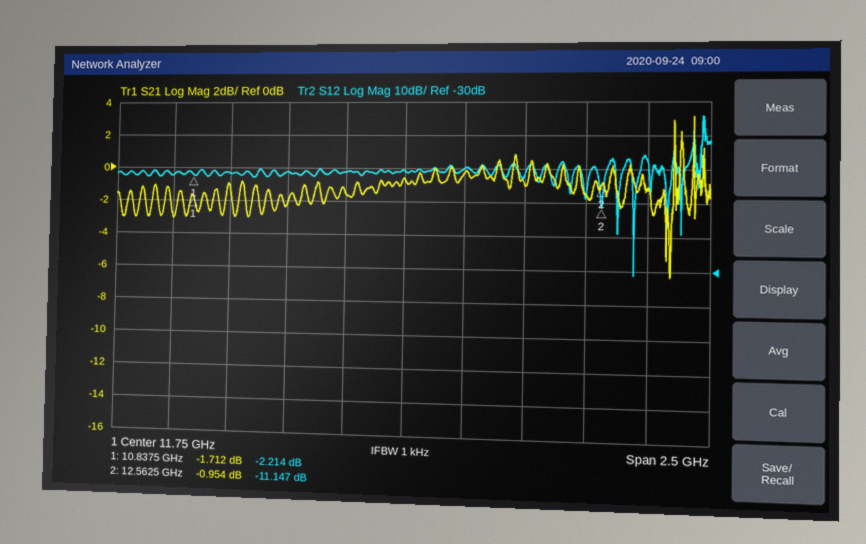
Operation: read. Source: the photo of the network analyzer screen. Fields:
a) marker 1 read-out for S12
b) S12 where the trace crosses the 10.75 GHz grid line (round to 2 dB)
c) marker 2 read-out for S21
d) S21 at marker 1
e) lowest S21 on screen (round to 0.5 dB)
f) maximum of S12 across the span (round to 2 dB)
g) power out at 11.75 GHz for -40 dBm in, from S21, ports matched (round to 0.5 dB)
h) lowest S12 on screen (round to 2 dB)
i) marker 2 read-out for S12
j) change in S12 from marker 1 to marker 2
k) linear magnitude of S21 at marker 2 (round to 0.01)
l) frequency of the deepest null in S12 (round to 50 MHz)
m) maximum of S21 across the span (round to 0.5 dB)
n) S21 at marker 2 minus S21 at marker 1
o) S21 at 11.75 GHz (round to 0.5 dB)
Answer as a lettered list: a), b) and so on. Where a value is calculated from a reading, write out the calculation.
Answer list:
a) -2.214 dB
b) -2 dB
c) -0.954 dB
d) -1.712 dB
e) -6.5 dB
f) 16 dB
g) -40 dBm + (-0.5 dB) = -40.5 dBm
h) -32 dB
i) -11.147 dB
j) -11.147 − (-2.214) = -8.933 dB
k) 10^(-0.954/20) ≈ 0.90
l) 12.70 GHz
m) 3.0 dB
n) -0.954 − (-1.712) = 0.758 dB
o) -0.5 dB
